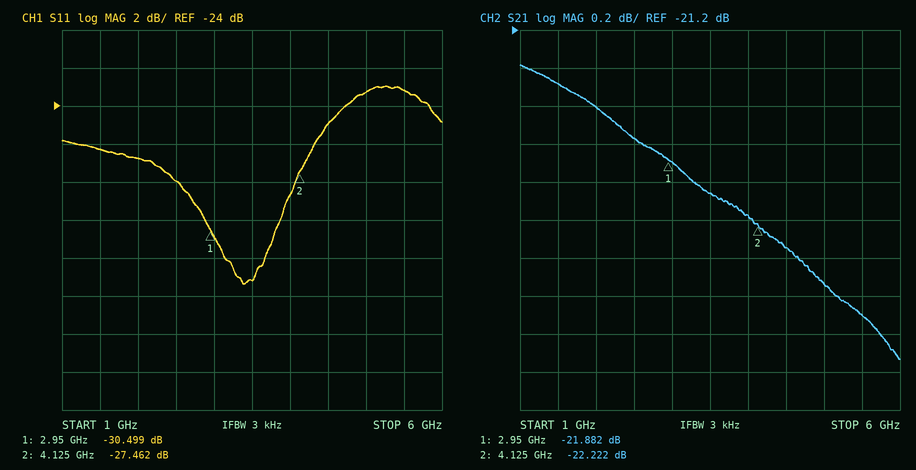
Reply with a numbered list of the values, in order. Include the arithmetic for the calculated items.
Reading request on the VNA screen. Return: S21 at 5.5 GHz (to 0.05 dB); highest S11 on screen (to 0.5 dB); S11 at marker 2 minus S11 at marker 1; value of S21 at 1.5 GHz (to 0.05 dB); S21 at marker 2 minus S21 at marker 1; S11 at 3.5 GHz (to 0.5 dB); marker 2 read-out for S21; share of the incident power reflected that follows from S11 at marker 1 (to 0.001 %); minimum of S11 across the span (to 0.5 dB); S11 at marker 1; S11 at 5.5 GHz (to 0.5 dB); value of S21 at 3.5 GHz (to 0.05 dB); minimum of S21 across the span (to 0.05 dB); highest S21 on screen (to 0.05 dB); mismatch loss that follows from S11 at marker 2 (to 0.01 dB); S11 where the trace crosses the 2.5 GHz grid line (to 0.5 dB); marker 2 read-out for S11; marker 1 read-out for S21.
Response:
1. -22.70 dB
2. -23.0 dB
3. -27.462 − (-30.499) = 3.037 dB
4. -21.50 dB
5. -22.222 − (-21.882) = -0.340 dB
6. -33.0 dB
7. -22.222 dB
8. 10^(-30.499/10) ≈ 0.089 %
9. -33.5 dB
10. -30.499 dB
11. -23.0 dB
12. -22.05 dB
13. -22.95 dB
14. -21.40 dB
15. −10 log10(1 − 10^(-27.462/10)) ≈ 0.01 dB
16. -28.0 dB
17. -27.462 dB
18. -21.882 dB
